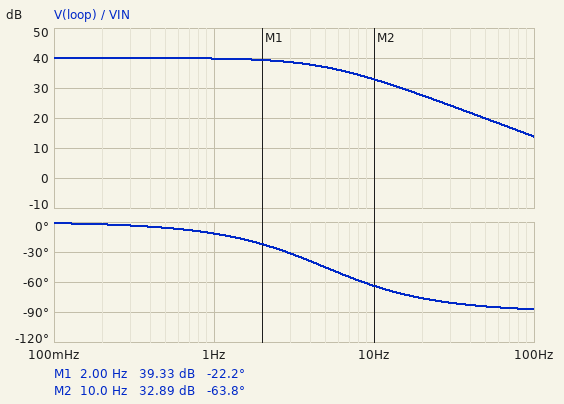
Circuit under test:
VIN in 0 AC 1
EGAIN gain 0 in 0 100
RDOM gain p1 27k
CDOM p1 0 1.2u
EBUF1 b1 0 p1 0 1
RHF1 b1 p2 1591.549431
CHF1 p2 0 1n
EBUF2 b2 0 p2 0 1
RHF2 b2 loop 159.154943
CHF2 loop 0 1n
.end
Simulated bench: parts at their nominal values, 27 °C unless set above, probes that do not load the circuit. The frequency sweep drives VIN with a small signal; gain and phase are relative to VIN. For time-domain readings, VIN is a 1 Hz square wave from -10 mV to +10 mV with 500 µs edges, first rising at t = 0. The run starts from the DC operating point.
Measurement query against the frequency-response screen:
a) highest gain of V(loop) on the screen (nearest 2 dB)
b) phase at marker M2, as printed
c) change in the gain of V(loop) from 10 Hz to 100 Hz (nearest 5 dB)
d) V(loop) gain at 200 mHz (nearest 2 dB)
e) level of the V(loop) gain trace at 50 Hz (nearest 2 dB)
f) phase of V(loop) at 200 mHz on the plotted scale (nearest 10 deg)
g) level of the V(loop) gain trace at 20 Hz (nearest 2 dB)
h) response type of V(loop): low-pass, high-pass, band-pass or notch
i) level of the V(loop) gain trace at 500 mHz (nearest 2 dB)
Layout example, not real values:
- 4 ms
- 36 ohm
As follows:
- 40 dB
- -63.8 deg
- -20 dB
- 40 dB
- 20 dB
- 0 deg
- 28 dB
- low-pass
- 40 dB
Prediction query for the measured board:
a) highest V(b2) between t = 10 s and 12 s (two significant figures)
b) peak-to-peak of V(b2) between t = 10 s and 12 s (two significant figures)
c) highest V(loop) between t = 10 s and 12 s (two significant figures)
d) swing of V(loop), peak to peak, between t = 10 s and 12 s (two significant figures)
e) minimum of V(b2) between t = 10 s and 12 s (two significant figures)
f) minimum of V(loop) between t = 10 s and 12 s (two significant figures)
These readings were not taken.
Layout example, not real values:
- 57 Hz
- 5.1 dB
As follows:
- 1.0 V
- 2.0 V
- 1.0 V
- 2.0 V
- -1.0 V
- -1.0 V
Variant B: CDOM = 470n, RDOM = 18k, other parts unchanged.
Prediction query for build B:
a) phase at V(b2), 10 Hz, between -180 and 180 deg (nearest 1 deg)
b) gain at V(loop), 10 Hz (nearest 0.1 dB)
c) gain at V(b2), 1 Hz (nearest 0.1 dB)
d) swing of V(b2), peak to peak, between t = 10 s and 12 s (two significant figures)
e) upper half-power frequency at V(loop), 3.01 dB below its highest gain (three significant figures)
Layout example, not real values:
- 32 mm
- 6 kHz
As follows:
- -28 deg
- 38.9 dB
- 40.0 dB
- 2.0 V
- 18.8 Hz
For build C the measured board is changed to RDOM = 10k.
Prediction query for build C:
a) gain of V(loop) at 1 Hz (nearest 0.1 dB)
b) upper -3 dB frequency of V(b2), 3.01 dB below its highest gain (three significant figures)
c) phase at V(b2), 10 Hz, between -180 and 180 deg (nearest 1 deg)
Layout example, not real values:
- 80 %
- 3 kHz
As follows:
- 40.0 dB
- 13.3 Hz
- -37 deg
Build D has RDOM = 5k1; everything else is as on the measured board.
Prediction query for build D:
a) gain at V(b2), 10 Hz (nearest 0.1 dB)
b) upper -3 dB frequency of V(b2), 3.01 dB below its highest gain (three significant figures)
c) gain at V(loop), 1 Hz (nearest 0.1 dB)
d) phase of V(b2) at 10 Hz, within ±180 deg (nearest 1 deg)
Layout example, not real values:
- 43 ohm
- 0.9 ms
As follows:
- 39.4 dB
- 26.0 Hz
- 40.0 dB
- -21 deg
